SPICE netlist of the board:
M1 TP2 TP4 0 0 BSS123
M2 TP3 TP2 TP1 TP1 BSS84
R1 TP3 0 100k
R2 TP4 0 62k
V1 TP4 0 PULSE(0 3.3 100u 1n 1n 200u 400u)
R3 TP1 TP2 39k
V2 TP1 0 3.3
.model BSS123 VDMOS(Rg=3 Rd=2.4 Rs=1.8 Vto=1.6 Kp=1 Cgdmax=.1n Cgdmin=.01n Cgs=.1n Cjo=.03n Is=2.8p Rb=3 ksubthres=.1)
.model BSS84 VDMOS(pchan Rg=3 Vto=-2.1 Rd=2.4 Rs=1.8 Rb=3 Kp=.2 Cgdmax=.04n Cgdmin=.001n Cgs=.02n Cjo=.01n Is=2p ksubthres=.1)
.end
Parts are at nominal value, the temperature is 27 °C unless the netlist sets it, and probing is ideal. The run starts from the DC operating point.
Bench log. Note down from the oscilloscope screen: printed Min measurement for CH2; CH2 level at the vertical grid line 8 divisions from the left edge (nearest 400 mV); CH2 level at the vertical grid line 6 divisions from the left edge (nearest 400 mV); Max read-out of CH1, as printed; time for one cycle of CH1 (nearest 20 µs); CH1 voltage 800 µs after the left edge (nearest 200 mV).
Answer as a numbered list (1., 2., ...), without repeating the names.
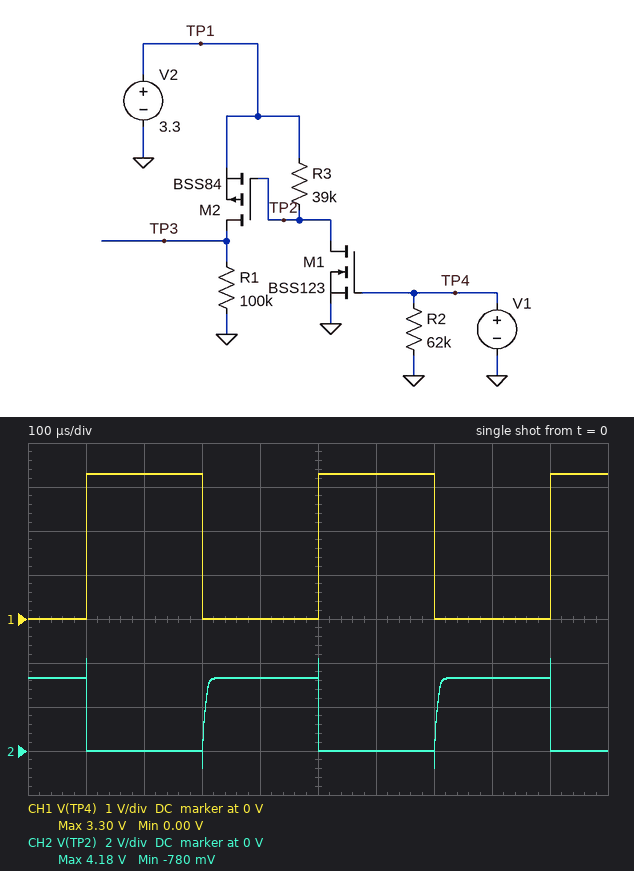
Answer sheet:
1. -780 mV
2. 3.2 V
3. 0 V
4. 3.30 V
5. 400 µs
6. 0 V
